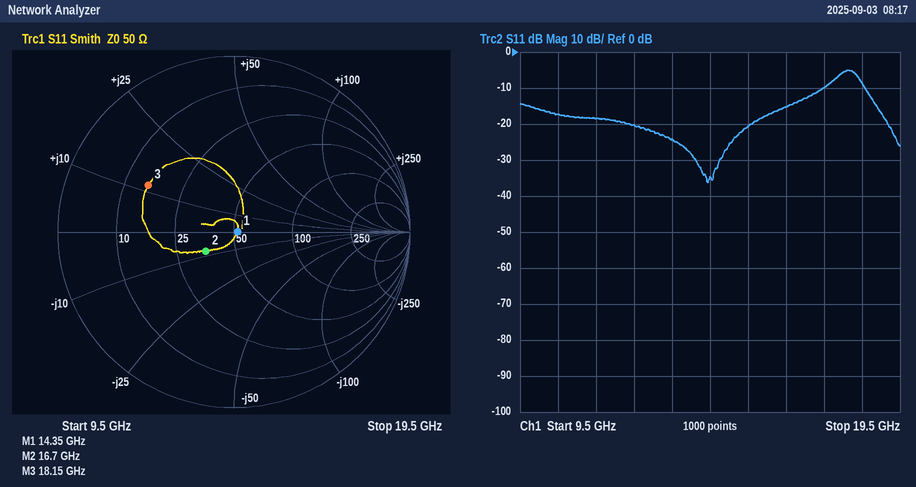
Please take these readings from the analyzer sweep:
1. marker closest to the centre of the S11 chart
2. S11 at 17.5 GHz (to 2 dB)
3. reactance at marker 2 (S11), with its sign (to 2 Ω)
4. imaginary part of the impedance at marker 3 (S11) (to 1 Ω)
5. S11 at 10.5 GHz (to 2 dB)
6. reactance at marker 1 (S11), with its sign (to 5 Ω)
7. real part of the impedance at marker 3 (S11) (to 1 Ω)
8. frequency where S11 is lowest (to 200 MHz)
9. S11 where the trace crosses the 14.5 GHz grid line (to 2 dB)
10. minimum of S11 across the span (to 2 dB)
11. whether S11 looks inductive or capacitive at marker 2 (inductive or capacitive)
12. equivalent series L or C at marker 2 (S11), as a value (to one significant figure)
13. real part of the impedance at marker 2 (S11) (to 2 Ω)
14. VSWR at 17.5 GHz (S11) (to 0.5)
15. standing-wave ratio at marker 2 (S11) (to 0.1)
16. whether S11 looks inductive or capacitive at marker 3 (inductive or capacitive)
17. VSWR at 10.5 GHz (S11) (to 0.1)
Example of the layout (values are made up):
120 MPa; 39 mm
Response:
marker 1; -10 dB; -8 Ω; +12 Ω; -18 dB; 0 Ω; 15 Ω; 14.4 GHz; -34 dB; -36 dB; capacitive; 1 pF; 36 Ω; 2.0; 1.5; inductive; 1.3
